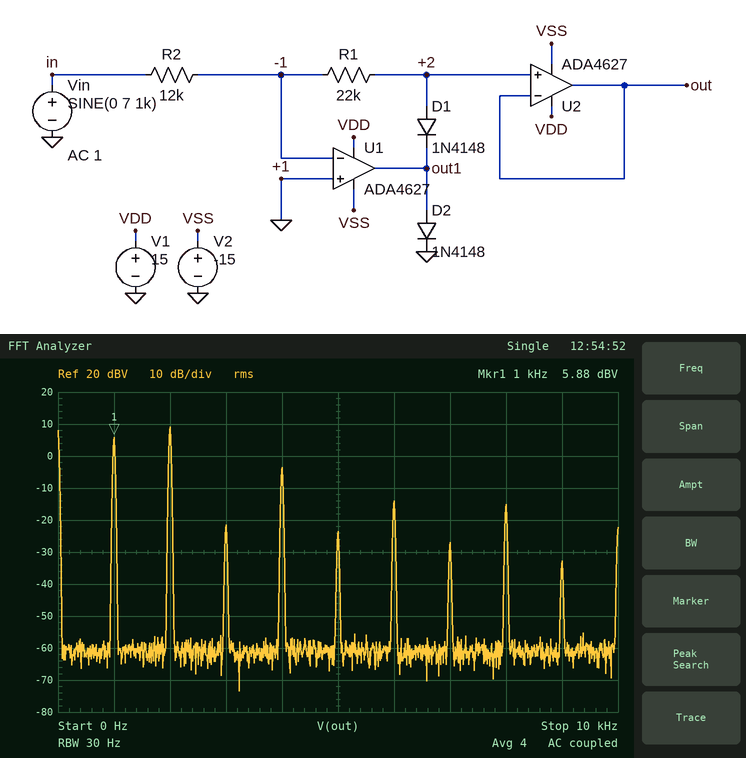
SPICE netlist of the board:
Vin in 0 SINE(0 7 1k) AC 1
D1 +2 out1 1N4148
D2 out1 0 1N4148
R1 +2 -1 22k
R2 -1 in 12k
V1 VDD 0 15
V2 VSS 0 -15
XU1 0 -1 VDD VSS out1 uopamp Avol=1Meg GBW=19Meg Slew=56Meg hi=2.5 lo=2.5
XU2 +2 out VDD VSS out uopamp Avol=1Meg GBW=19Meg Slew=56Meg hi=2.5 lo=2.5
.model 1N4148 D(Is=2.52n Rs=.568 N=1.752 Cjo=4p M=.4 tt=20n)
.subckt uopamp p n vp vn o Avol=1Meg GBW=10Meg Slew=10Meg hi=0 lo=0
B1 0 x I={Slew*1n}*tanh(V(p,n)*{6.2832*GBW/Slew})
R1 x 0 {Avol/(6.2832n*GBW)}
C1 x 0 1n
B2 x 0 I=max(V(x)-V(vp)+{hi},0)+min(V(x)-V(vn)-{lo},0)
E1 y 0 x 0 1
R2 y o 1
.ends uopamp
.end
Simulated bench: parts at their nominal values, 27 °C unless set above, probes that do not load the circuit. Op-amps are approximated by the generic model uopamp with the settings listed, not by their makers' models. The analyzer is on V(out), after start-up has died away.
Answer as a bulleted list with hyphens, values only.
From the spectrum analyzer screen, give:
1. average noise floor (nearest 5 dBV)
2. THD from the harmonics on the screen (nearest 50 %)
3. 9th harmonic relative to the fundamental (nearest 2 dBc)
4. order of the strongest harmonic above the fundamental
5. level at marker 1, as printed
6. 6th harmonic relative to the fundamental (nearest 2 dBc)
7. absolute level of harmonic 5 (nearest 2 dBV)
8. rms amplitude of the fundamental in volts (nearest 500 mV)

- -60 dBV
- 150 %
- -38 dBc
- 2
- 5.88 dBV
- -20 dBc
- -24 dBV
- 2.0 V
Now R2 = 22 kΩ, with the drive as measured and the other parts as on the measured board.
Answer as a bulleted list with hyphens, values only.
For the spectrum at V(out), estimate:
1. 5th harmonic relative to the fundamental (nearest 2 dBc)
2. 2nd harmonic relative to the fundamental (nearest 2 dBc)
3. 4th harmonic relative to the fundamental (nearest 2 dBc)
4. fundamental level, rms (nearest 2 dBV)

- -8 dBc
- 64 dBc
- 50 dBc
- -56 dBV
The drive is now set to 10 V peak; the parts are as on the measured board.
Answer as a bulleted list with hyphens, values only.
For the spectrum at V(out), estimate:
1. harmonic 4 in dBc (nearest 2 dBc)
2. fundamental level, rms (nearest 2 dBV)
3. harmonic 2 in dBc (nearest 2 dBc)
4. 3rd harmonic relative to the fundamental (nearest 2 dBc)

- -2 dBc
- 4 dBV
- 6 dBc
- -6 dBc
